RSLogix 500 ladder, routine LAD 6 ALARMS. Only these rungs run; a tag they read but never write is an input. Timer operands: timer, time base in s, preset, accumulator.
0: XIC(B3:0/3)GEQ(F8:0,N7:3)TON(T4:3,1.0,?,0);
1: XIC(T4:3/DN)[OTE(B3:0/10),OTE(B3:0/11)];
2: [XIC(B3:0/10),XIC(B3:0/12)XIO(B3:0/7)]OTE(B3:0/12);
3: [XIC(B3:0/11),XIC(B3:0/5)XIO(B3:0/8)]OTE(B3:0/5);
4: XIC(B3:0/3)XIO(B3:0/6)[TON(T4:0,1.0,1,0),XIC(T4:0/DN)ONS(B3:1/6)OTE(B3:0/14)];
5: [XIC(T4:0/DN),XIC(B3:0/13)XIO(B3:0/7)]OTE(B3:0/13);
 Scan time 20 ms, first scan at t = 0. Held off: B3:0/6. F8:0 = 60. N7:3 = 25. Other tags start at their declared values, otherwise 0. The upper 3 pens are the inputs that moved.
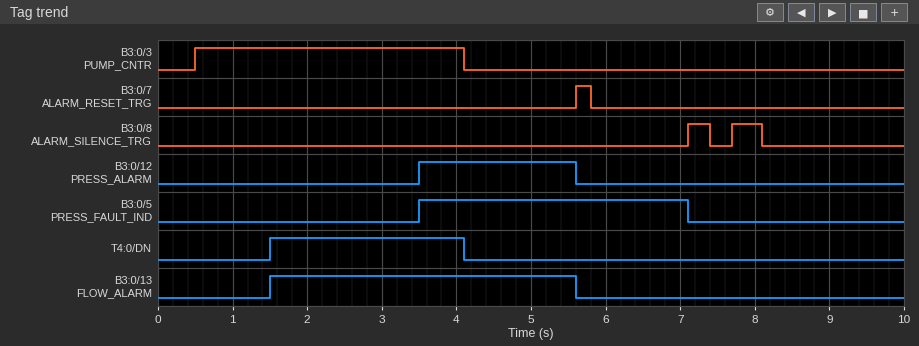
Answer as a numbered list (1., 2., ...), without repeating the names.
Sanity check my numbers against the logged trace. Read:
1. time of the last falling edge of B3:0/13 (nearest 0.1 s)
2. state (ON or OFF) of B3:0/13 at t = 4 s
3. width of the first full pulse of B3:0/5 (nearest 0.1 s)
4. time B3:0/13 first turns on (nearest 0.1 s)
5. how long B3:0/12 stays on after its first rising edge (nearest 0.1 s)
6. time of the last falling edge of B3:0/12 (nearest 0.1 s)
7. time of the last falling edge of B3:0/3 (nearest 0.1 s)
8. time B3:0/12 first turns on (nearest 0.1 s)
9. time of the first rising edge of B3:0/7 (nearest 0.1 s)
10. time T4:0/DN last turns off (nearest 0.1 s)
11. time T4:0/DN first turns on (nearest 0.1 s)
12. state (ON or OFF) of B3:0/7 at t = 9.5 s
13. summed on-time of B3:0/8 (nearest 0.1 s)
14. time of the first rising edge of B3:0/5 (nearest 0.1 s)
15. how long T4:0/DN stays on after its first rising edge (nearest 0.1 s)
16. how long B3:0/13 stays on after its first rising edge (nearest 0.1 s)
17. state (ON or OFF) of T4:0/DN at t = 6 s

1. 5.6 s
2. ON
3. 3.6 s
4. 1.5 s
5. 2.1 s
6. 5.6 s
7. 4.1 s
8. 3.5 s
9. 5.6 s
10. 4.1 s
11. 1.5 s
12. OFF
13. 0.7 s
14. 3.5 s
15. 2.6 s
16. 4.1 s
17. OFF
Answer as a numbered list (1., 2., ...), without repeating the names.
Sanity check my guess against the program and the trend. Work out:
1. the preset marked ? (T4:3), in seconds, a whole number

1. 3 s
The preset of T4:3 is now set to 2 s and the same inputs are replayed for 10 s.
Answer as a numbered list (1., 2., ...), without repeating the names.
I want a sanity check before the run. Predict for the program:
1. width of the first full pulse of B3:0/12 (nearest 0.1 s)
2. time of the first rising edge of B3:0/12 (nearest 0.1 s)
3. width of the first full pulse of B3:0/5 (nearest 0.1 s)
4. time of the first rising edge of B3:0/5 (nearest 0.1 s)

1. 3.1 s
2. 2.5 s
3. 4.6 s
4. 2.5 s
